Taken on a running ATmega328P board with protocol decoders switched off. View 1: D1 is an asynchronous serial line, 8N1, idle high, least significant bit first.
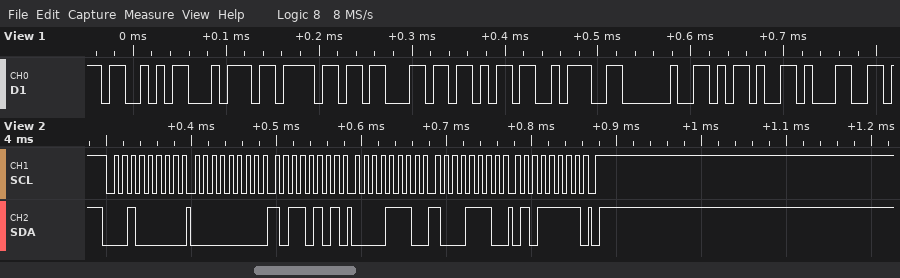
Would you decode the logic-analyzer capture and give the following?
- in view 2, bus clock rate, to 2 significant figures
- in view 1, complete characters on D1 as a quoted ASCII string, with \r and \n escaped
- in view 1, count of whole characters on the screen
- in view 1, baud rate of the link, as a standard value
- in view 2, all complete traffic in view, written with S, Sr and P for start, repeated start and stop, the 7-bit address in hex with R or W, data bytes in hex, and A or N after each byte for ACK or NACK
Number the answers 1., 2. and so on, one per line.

1. 100 kHz
2. "Stock: -1"
3. 9
4. 115200 baud
5. S 10W A 00 A B5 A 0E A 8E A 5F A P
